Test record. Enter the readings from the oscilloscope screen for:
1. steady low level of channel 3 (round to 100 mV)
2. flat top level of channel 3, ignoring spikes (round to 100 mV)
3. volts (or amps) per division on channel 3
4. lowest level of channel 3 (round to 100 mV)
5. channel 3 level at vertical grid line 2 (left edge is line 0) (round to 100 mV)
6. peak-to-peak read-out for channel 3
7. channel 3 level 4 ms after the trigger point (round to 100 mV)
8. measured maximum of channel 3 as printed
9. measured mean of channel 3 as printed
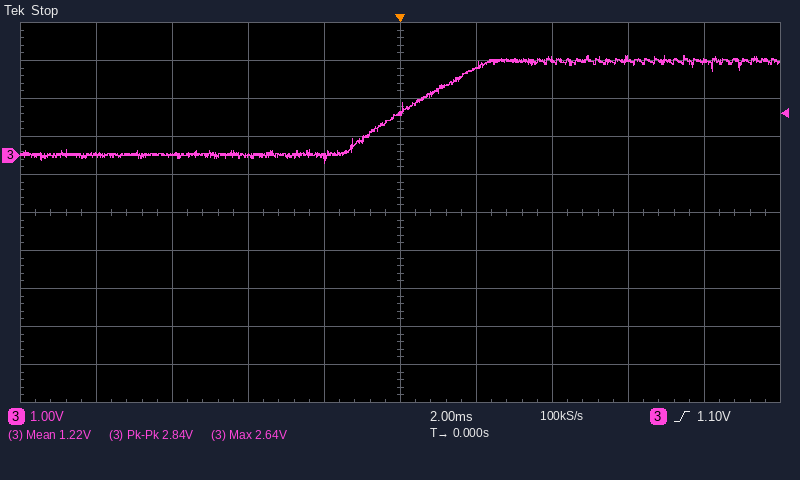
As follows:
0.0 V
2.5 V
1 V
-200 mV
0.0 V
2.84 V
2.5 V
2.64 V
1.22 V
